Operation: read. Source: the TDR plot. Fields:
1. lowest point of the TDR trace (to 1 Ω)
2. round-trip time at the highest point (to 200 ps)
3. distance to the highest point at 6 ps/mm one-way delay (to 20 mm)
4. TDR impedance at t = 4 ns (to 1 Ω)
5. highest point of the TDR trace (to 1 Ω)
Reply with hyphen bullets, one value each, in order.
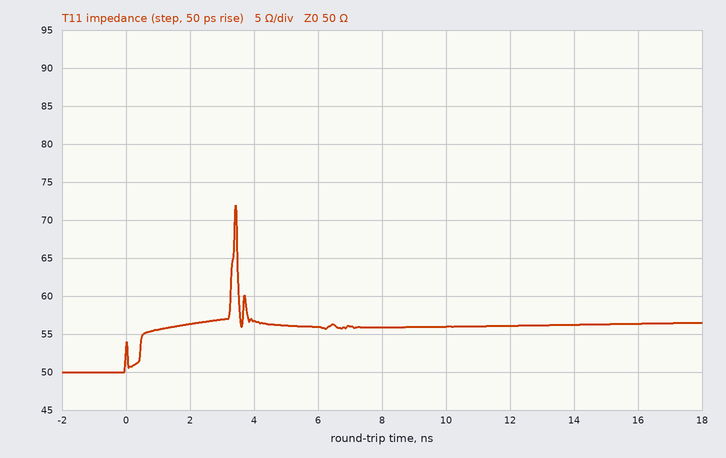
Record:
- 50 Ω
- 3.4 ns
- 280 mm
- 57 Ω
- 72 Ω
